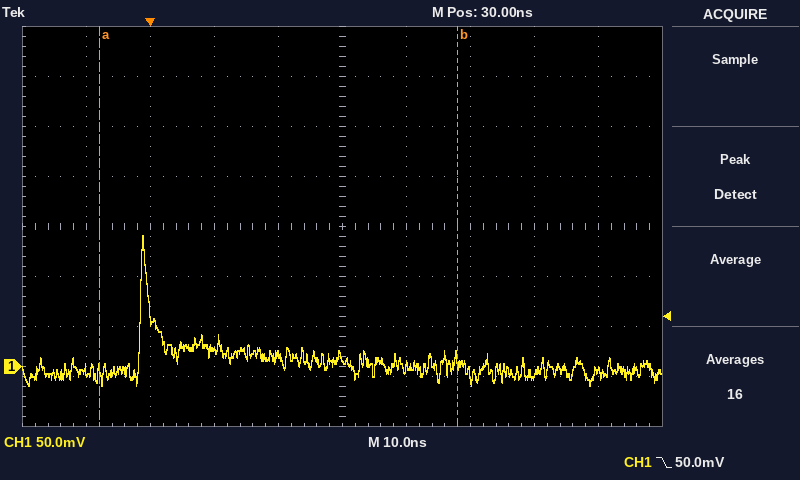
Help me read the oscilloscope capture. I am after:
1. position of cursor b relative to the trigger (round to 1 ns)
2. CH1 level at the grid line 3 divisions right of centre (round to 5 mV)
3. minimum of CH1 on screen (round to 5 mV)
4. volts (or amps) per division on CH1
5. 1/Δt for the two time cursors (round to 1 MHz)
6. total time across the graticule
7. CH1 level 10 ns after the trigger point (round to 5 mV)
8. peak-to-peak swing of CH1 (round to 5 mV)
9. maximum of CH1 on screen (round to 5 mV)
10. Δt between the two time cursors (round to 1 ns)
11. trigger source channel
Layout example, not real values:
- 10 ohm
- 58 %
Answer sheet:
- +48 ns
- -10 mV
- -20 mV
- 50 mV
- 18 MHz
- 100 ns
- 15 mV
- 150 mV
- 130 mV
- 56 ns
- CH1
